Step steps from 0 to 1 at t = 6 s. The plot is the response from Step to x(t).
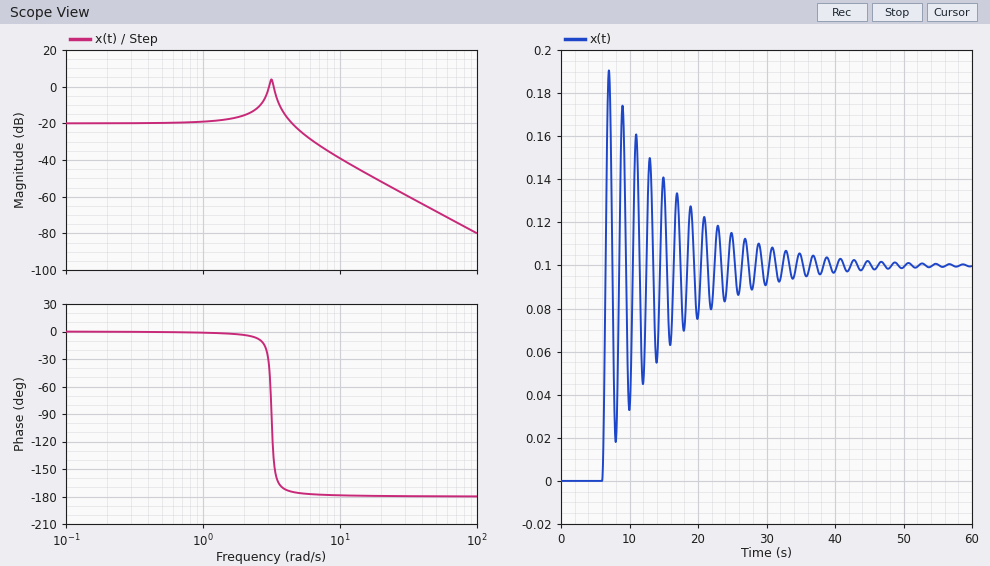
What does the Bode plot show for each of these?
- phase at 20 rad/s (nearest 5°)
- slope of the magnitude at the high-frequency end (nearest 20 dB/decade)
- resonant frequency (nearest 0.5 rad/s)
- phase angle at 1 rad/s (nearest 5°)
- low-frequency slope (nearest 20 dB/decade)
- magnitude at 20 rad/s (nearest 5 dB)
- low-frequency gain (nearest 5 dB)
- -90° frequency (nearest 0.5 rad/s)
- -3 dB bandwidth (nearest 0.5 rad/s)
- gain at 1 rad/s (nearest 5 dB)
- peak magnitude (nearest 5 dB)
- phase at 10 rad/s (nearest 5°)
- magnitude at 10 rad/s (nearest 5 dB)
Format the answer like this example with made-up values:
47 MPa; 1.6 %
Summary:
-180°; -40 dB/decade; 3.0 rad/s; 0°; 0 dB/decade; -50 dB; -20 dB; 3.0 rad/s; 5.0 rad/s; -20 dB; 5 dB; -180°; -40 dB
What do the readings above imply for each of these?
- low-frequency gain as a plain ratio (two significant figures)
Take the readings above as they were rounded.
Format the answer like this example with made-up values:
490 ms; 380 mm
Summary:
0.10
